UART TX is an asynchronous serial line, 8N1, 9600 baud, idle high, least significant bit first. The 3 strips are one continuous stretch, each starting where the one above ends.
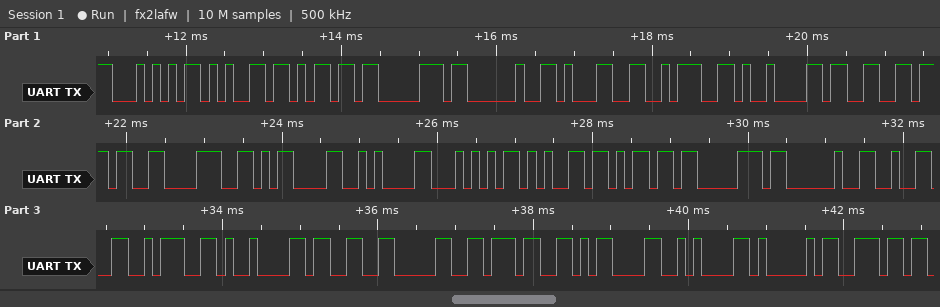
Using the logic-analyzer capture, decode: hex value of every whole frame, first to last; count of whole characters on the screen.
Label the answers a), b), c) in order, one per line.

a) 0x54 0x65 0x6D 0x70 0x20 0x31 0x3A 0x09 0x33 0x37 0x38 0x0D 0x0A 0x54 0x65 0x6D 0x70 0x20 0x32 0x3A 0x09 0x33 0x30 0x37 0x0D 0x0A 0x41 0x6E
b) 28
